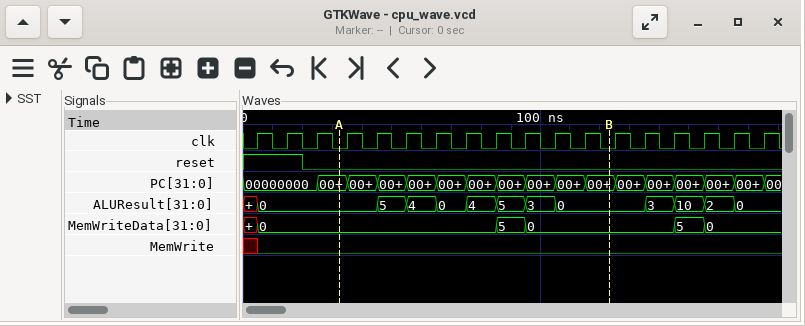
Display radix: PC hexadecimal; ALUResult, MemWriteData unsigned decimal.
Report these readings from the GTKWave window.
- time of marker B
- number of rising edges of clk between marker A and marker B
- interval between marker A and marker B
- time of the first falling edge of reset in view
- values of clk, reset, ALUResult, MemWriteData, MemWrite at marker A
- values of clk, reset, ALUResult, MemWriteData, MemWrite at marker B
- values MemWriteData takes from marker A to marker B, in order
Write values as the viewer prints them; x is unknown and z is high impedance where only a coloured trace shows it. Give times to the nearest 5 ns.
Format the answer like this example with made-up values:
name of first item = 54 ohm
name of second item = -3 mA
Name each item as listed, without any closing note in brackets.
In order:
time of marker B = 125 ns
number of rising edges of clk between marker A and marker B = 9
interval between marker A and marker B = 90 ns
time of the first falling edge of reset in view = 20 ns
values of clk, reset, ALUResult, MemWriteData, MemWrite at marker A = clk=0, reset=0, ALUResult=0, MemWriteData=0, MemWrite=0
values of clk, reset, ALUResult, MemWriteData, MemWrite at marker B = clk=0, reset=0, ALUResult=0, MemWriteData=0, MemWrite=0
values MemWriteData takes from marker A to marker B, in order = 0, 5, 0
